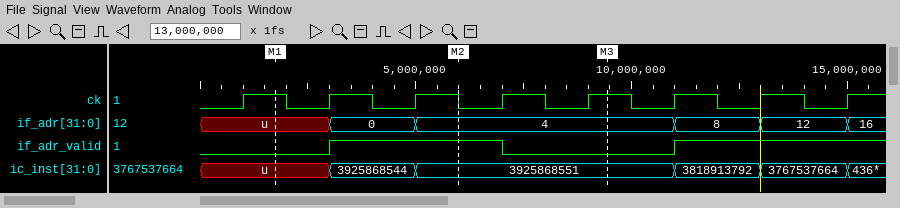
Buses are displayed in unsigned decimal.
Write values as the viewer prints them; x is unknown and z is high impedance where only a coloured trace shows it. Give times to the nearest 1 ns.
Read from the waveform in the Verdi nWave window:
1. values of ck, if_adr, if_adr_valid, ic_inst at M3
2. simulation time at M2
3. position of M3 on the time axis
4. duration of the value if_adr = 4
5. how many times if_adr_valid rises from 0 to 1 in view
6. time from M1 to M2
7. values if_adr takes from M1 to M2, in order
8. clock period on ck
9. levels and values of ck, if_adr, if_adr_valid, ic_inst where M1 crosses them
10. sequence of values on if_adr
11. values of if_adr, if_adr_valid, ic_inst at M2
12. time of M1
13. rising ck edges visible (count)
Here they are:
ck=1, if_adr=4, if_adr_valid=0, ic_inst=3925868551
6 ns
9 ns
6 ns
2
4 ns
u, 0, 4
2 ns
ck=1, if_adr=u, if_adr_valid=0, ic_inst=u
u, 0, 4, 8, 12, 16
if_adr=4, if_adr_valid=1, ic_inst=3925868551
2 ns
8
